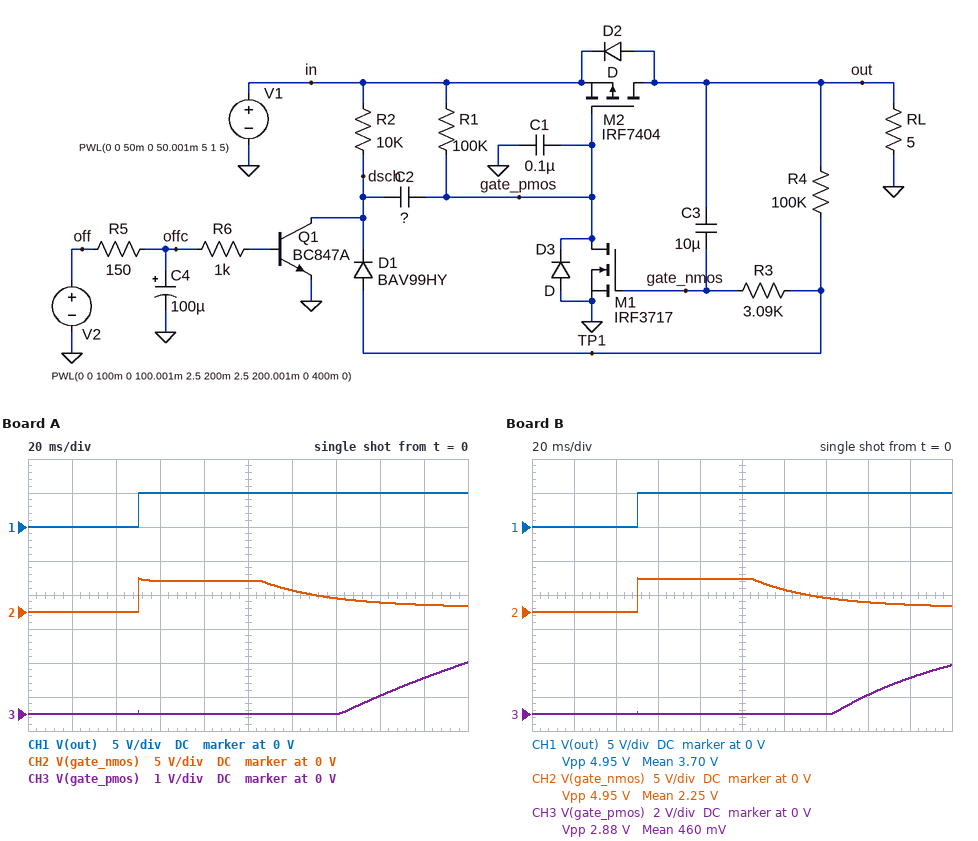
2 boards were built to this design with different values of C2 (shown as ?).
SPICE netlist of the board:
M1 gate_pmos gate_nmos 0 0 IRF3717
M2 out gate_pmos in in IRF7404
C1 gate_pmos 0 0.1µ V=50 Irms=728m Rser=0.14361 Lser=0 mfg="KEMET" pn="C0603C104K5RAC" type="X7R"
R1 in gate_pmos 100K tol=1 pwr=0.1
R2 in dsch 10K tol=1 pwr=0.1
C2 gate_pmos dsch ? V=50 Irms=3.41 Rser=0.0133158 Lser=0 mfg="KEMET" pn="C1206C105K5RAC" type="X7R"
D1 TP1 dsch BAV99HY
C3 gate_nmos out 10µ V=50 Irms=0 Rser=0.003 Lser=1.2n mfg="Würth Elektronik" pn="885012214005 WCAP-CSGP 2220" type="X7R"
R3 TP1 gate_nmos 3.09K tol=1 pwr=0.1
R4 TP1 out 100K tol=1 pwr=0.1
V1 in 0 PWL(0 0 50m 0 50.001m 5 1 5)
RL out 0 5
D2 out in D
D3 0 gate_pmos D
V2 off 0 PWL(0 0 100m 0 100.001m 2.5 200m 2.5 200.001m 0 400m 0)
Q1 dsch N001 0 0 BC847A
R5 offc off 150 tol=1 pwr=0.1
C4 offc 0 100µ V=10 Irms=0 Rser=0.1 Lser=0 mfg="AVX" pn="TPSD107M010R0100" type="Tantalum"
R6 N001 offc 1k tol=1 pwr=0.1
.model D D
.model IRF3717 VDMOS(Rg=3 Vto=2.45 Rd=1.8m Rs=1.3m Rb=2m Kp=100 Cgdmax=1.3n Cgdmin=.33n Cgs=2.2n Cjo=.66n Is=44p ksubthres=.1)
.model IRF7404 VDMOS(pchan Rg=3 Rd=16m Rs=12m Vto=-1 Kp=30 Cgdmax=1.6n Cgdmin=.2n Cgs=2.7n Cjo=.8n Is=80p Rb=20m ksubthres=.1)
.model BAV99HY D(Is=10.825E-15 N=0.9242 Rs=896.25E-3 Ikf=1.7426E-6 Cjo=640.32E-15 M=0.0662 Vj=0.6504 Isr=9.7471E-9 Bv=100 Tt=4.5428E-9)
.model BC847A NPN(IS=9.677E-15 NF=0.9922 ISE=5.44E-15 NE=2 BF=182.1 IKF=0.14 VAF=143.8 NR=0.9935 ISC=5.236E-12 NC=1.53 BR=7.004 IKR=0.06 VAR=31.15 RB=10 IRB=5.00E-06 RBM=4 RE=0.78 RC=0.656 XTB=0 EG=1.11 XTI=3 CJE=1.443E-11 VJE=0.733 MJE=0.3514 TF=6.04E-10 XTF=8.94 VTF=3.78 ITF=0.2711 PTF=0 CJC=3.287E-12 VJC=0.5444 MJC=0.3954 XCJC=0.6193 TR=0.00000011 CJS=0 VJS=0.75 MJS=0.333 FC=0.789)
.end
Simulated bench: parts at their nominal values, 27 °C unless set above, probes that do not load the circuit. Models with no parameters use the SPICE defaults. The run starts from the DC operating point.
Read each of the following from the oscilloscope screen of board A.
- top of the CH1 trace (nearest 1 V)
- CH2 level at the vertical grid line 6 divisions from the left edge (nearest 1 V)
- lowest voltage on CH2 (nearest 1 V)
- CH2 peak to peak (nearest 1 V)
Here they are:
5 V
3 V
0 V
5 V
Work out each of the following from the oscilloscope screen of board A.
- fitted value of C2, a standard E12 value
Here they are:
1.5 µF
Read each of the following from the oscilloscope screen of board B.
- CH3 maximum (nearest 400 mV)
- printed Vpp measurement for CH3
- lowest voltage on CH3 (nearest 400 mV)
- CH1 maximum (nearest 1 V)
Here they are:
2.8 V
2.88 V
0 V
5 V
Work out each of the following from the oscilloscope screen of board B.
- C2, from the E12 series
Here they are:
560 nF
